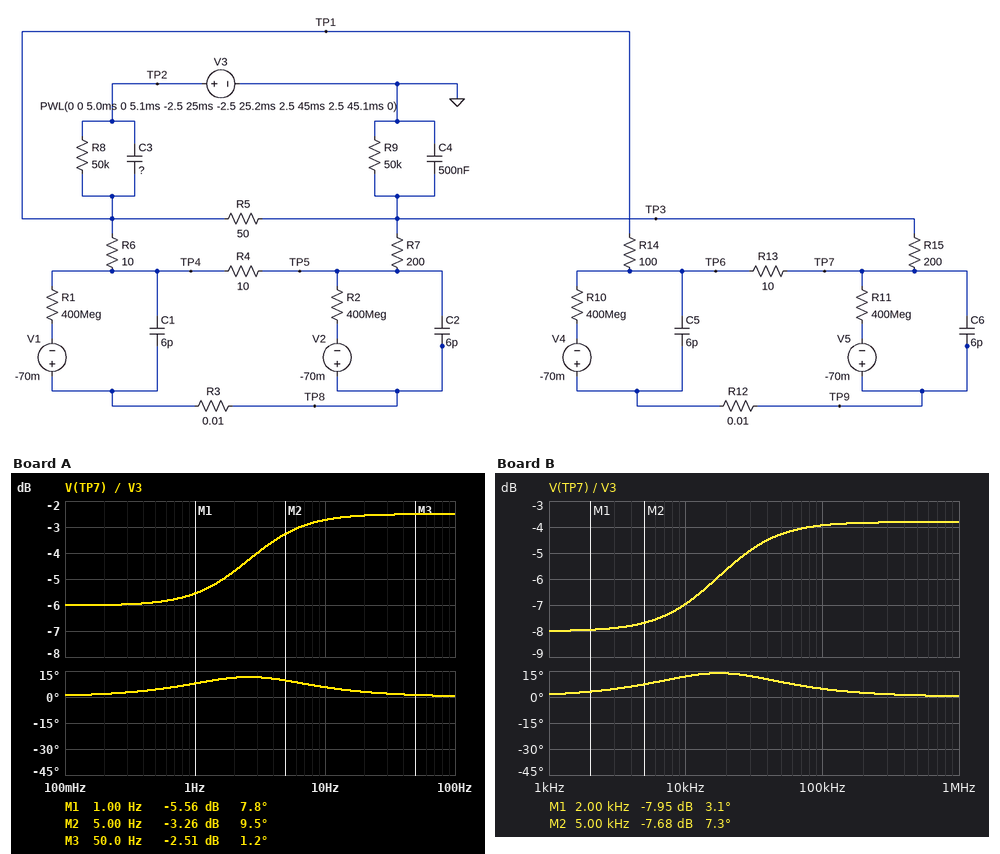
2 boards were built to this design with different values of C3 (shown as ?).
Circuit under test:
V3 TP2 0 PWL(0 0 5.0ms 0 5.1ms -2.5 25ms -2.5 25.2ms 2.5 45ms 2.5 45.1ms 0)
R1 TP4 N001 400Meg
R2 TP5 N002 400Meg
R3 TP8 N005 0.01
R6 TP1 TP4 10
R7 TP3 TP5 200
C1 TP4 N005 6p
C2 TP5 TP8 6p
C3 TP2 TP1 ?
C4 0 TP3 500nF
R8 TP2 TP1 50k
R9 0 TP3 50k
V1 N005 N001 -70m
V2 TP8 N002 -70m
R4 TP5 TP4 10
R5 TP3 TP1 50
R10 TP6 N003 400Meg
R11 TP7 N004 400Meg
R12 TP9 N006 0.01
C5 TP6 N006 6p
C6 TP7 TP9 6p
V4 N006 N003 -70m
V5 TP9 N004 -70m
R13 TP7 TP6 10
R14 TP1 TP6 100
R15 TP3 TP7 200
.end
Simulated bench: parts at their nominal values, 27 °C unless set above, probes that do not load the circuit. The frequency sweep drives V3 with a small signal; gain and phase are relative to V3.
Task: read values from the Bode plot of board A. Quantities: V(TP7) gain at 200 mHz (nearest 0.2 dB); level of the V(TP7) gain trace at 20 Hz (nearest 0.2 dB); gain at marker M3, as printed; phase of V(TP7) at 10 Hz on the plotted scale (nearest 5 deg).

-6.0 dB
-2.6 dB
-2.51 dB
5 deg
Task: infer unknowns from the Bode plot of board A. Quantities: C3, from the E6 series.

1.5 µF
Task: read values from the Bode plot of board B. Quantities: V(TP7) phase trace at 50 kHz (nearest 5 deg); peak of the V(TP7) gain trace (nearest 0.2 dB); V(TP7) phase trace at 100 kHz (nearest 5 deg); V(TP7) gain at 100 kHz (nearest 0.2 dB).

10 deg
-3.8 dB
5 deg
-4.0 dB
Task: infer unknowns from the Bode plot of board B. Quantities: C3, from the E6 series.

330 nF
